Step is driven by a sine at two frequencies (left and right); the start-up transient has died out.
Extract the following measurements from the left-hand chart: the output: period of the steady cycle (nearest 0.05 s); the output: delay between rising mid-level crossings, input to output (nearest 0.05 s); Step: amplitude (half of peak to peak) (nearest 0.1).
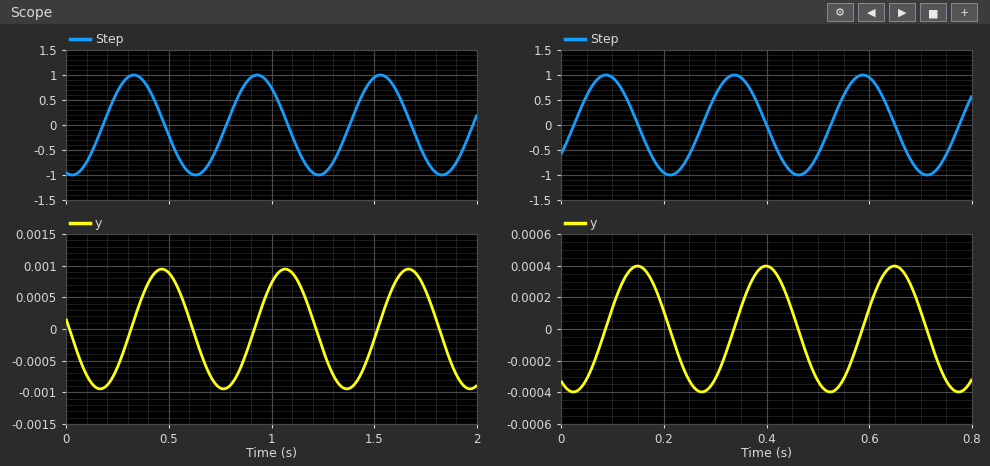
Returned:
0.60 s
0.15 s
1.0
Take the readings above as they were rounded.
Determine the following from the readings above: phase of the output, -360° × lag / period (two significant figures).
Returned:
-90°
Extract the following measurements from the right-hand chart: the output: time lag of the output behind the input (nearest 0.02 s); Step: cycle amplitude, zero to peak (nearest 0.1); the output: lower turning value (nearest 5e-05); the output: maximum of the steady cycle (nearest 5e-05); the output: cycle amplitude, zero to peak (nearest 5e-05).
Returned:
0.06 s
1.0
-0.00040
0.00040
0.00040
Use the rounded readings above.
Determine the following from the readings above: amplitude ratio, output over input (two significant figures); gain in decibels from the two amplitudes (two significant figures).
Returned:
0.00040
-68 dB
